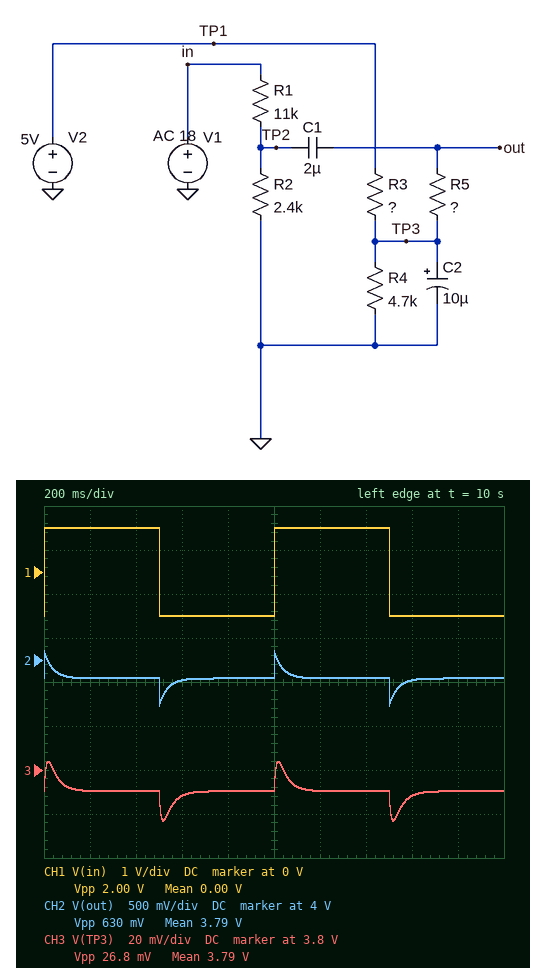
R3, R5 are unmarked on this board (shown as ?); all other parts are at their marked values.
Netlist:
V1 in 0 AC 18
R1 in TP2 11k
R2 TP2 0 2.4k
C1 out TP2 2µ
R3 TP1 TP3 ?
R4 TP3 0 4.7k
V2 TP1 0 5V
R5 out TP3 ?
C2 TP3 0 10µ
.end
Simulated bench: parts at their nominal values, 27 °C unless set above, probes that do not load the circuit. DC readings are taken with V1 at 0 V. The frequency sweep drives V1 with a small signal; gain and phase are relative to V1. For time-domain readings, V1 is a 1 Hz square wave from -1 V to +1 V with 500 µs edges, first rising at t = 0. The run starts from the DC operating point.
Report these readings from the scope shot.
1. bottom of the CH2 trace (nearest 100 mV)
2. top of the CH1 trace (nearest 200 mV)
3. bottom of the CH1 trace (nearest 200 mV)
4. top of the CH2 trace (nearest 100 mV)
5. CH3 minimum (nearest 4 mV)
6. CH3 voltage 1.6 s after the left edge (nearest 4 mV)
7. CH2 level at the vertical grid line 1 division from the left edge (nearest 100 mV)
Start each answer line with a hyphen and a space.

- 3.5 V
- 1.0 V
- -1.0 V
- 4.1 V
- 3.776 V
- 3.788 V
- 3.8 V
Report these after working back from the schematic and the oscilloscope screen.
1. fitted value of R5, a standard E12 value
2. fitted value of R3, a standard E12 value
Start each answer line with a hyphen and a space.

- 15 kΩ
- 1.5 kΩ
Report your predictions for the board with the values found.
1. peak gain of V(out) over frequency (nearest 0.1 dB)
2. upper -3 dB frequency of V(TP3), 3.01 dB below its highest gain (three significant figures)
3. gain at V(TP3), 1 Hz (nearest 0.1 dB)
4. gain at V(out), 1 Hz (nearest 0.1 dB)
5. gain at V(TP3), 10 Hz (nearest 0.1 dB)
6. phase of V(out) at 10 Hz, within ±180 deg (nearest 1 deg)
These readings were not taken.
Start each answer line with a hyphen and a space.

- -16.0 dB
- 22.5 Hz
- -52.1 dB
- -29.0 dB
- -41.5 dB
- 24 deg
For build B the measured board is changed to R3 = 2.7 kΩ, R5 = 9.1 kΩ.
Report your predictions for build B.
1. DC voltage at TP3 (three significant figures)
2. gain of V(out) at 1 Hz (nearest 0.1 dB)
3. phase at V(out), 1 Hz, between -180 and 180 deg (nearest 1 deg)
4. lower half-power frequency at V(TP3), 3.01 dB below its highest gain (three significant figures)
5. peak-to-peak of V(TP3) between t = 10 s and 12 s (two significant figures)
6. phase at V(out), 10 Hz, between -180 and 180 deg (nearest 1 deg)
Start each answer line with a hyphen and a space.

- 3.18 V
- -32.4 dB
- 80 deg
- 3.17 Hz
- 44 mV
- 32 deg
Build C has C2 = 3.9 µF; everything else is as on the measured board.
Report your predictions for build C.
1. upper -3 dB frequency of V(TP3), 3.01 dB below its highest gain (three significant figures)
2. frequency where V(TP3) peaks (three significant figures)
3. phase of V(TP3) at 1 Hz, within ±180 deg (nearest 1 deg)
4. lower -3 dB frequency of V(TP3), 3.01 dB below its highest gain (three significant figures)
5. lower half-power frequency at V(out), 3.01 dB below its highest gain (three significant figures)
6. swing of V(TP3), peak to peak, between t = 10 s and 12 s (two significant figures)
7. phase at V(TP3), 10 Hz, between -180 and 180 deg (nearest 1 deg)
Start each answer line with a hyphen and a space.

- 46.6 Hz
- 13.0 Hz
- 76 deg
- 3.61 Hz
- 4.36 Hz
- 34 mV
- 9 deg
